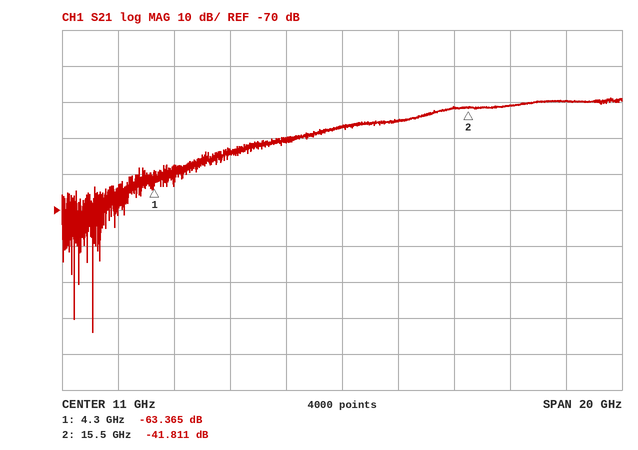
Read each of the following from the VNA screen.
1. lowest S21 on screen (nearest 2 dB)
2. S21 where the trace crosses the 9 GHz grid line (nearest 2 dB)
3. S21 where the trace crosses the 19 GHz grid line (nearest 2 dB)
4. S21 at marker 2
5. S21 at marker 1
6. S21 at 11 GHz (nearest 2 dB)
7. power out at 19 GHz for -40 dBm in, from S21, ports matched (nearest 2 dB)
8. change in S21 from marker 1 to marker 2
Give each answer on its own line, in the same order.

-104 dB
-50 dB
-40 dB
-41.811 dB
-63.365 dB
-46 dB
-80 dBm
21.554 dB
